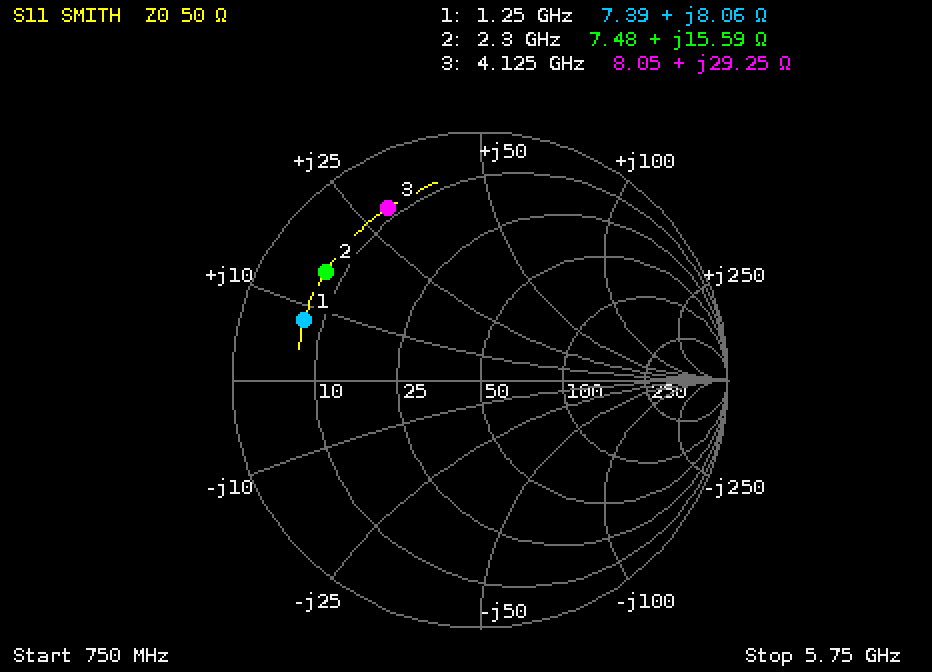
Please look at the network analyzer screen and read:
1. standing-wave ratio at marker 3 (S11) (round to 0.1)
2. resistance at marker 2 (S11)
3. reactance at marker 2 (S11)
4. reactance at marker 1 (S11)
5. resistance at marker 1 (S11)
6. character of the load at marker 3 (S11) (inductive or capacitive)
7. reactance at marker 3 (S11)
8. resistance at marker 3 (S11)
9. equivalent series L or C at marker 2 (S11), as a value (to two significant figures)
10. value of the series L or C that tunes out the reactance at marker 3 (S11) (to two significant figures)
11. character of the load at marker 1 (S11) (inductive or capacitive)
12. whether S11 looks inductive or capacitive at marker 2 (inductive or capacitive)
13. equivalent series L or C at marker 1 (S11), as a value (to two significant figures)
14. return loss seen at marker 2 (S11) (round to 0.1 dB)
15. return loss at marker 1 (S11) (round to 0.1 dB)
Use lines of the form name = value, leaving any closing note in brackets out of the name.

standing-wave ratio at marker 3 (S11) = 8.4
resistance at marker 2 = 7.48 Ω
reactance at marker 2 = +15.59 Ω
reactance at marker 1 = +8.06 Ω
resistance at marker 1 = 7.39 Ω
character of the load at marker 3 (S11) = inductive
reactance at marker 3 = +29.25 Ω
resistance at marker 3 = 8.05 Ω
equivalent series L or C at marker 2 (S11), as a value = 1.1 nH
value of the series L or C that tunes out the reactance at marker 3 (S11) = 1.3 pF
character of the load at marker 1 (S11) = inductive
whether S11 looks inductive or capacitive at marker 2 = inductive
equivalent series L or C at marker 1 (S11), as a value = 1.0 nH
return loss seen at marker 2 (S11) = 2.4 dB
return loss at marker 1 (S11) = 2.5 dB
